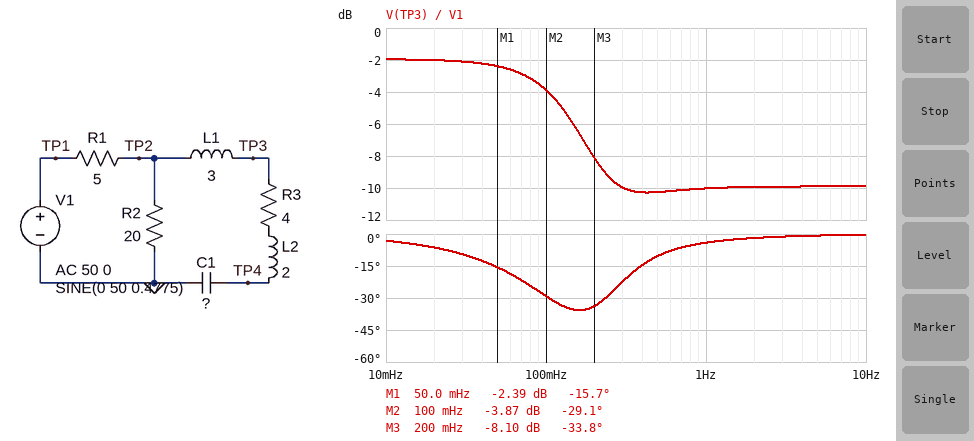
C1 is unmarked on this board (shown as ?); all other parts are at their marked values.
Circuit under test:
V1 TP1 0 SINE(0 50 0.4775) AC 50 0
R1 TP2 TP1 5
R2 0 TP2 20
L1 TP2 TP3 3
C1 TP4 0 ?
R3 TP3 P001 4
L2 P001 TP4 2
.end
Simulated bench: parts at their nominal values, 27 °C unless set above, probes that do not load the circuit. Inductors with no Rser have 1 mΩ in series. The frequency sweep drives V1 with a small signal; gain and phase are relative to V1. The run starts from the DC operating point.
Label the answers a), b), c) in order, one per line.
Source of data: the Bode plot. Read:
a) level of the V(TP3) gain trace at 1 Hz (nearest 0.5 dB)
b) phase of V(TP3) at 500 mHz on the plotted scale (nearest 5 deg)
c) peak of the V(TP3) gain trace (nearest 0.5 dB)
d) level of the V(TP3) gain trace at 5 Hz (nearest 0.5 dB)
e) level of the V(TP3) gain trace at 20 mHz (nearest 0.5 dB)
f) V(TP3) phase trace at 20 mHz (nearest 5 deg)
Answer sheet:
a) -10.0 dB
b) -10 deg
c) -2.0 dB
d) -10.0 dB
e) -2.0 dB
f) -5 deg
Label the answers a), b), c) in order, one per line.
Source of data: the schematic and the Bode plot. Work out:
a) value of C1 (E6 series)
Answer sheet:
a) 220 mF
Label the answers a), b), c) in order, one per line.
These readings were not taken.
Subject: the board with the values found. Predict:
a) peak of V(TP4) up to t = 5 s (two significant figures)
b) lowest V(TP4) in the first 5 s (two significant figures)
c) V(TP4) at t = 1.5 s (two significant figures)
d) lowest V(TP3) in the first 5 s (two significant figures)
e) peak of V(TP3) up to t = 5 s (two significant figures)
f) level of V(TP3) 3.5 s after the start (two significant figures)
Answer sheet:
a) 9.2 V
b) -3.5 V
c) 8.8 V
d) -15 V
e) 19 V
f) -11 V
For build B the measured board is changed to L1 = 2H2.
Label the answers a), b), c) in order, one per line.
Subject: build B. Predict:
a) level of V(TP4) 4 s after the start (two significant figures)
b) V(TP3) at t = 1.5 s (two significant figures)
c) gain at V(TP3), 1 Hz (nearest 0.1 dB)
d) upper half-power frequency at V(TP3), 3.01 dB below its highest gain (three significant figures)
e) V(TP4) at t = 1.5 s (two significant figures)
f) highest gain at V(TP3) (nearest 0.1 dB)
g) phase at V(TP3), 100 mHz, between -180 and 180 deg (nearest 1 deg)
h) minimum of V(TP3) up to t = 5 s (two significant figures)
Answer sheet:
a) 430 mV
b) -14 V
c) -8.6 dB
d) 121 mHz
e) 9.0 V
f) -1.9 dB
g) -26 deg
h) -17 V
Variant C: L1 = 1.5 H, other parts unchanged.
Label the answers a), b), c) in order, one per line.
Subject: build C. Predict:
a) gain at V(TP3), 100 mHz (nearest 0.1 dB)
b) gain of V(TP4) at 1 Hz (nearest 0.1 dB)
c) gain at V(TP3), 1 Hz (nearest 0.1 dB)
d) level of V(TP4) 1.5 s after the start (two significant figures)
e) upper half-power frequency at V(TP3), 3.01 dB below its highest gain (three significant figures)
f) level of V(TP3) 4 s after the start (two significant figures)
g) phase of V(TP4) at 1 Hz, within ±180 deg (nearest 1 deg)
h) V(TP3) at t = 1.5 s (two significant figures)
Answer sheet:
a) -4.3 dB
b) -31.9 dB
c) -7.1 dB
d) 9.1 V
e) 116 mHz
f) -10 V
g) -159 deg
h) -17 V
